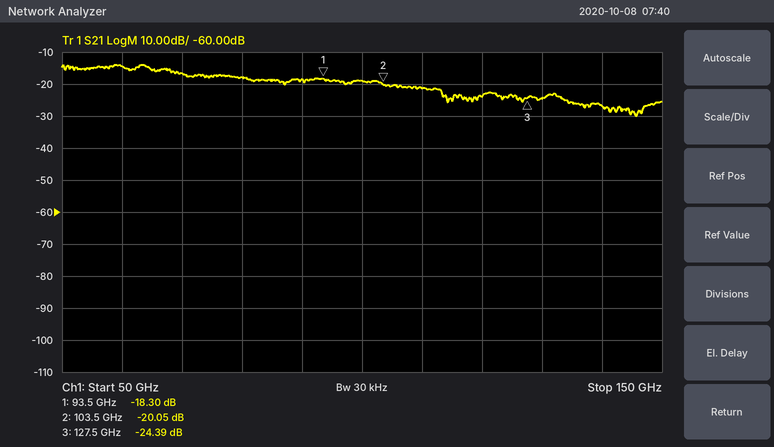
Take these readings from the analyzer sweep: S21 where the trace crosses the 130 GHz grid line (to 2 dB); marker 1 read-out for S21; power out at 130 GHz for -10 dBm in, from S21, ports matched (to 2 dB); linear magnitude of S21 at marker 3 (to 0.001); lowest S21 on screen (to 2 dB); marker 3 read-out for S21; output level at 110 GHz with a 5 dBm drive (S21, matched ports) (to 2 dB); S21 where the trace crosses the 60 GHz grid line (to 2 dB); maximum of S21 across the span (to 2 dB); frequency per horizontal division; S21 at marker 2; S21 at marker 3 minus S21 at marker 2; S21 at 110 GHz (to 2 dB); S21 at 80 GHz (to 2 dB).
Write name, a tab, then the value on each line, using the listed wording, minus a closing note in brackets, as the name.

S21 where the trace crosses the 130 GHz grid line	-24 dB
marker 1 read-out for S21	-18.30 dB
power out at 130 GHz for -10 dBm in, from S21, ports matched	-34 dBm
linear magnitude of S21 at marker 3	0.060
lowest S21 on screen	-30 dB
marker 3 read-out for S21	-24.39 dB
output level at 110 GHz with a 5 dBm drive (S21, matched ports)	-16 dBm
S21 where the trace crosses the 60 GHz grid line	-14 dB
maximum of S21 across the span	-14 dB
frequency per horizontal division	10 GHz
S21 at marker 2	-20.05 dB
S21 at marker 3 minus S21 at marker 2	-4.34 dB
S21 at 110 GHz	-22 dB
S21 at 80 GHz	-18 dB
